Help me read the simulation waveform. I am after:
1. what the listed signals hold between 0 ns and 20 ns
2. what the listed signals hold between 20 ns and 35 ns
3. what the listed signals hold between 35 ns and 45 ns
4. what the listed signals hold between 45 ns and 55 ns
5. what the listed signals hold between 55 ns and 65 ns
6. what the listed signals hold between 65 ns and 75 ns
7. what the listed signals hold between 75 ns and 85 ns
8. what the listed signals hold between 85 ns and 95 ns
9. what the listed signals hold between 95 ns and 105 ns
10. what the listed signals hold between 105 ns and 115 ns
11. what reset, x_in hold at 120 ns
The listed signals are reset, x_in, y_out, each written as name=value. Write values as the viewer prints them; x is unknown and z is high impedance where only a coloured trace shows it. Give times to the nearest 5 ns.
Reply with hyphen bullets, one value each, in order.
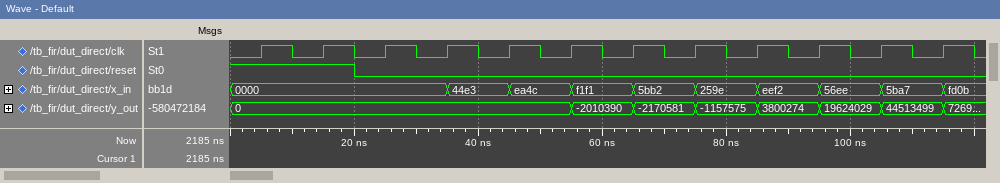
- reset=1, x_in=0000, y_out=0
- reset=0, x_in=0000, y_out=0
- reset=0, x_in=44e3, y_out=0
- reset=0, x_in=ea4c, y_out=0
- reset=0, x_in=f1f1, y_out=-2010390
- reset=0, x_in=5bb2, y_out=-2170581
- reset=0, x_in=259e, y_out=-1157575
- reset=0, x_in=eef2, y_out=3800274
- reset=0, x_in=56ee, y_out=19624029
- reset=0, x_in=5ba7, y_out=44513499
- reset=0, x_in=fd0b
